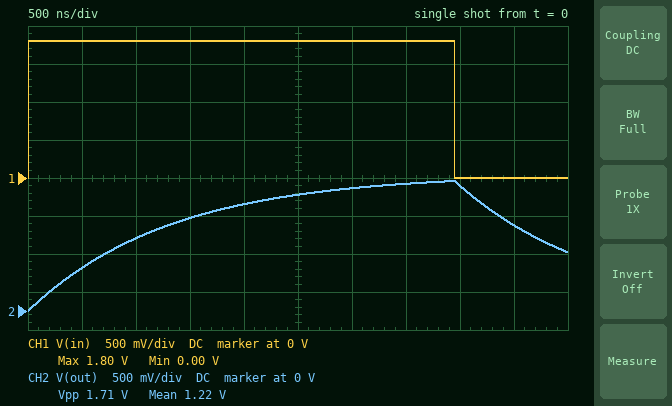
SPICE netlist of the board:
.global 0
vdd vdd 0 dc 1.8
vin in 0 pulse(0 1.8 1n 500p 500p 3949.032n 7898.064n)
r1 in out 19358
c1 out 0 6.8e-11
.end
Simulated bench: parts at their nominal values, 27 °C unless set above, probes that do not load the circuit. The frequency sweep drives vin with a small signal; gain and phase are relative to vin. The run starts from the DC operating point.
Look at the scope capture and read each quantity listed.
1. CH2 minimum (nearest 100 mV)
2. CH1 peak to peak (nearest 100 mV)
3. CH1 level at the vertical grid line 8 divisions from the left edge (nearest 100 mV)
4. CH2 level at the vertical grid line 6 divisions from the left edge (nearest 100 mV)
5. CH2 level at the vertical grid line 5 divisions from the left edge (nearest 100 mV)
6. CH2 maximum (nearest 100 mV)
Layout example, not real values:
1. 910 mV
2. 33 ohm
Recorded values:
1. 0 V
2. 1.8 V
3. 0 V
4. 1.6 V
5. 1.5 V
6. 1.7 V
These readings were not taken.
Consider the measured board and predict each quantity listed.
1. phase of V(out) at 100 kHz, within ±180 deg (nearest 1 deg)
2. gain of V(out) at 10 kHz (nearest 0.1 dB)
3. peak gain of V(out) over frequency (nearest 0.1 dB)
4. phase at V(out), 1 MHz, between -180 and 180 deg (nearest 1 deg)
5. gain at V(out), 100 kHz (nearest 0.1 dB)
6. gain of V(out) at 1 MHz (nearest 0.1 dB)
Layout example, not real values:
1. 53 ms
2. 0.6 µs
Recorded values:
1. -40 deg
2. 0 dB
3. 0 dB
4. -83 deg
5. -2.3 dB
6. -18.4 dB
